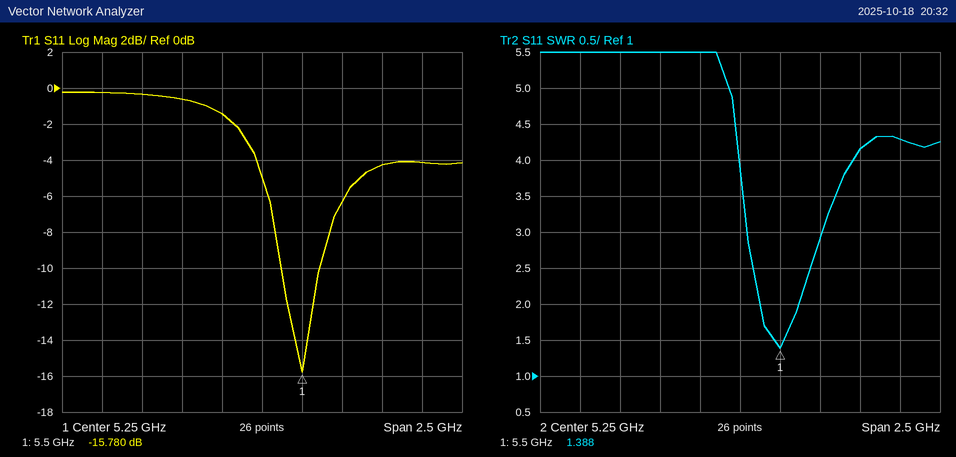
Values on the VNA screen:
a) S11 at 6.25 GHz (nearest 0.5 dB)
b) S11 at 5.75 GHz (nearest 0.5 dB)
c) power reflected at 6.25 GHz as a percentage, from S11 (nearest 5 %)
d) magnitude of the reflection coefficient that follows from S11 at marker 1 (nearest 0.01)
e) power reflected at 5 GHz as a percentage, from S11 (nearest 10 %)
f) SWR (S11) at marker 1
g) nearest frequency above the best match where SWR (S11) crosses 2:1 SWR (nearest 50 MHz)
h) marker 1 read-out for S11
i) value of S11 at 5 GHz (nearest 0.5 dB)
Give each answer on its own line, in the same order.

-4.0 dB
-6.5 dB
40 %
0.16
70 %
1.388
5.60 GHz
-15.780 dB
-1.5 dB
